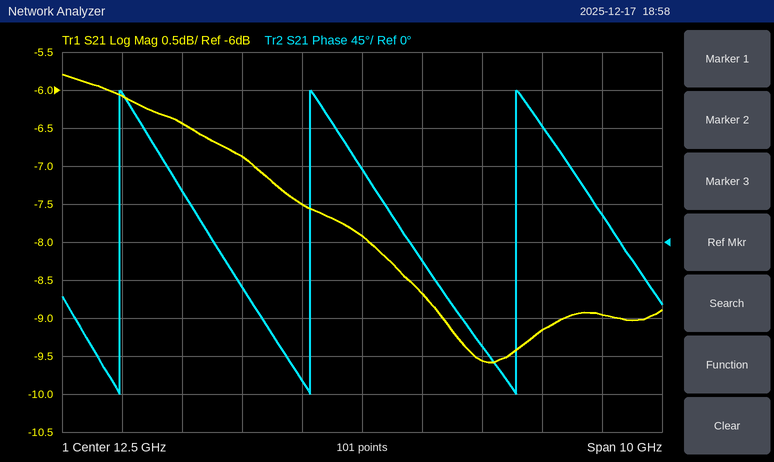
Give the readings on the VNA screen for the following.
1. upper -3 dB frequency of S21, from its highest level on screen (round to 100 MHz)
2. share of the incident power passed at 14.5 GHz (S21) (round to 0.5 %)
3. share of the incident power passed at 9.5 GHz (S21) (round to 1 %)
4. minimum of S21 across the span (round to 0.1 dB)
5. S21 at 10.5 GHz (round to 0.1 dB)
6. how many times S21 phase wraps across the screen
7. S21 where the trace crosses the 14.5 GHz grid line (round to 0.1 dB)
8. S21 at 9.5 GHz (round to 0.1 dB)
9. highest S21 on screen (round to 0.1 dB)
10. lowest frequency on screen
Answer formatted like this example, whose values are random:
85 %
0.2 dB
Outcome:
13.6 GHz
11.0 %
23 %
-9.6 dB
-6.9 dB
3
-9.6 dB
-6.4 dB
-5.8 dB
7.5 GHz
